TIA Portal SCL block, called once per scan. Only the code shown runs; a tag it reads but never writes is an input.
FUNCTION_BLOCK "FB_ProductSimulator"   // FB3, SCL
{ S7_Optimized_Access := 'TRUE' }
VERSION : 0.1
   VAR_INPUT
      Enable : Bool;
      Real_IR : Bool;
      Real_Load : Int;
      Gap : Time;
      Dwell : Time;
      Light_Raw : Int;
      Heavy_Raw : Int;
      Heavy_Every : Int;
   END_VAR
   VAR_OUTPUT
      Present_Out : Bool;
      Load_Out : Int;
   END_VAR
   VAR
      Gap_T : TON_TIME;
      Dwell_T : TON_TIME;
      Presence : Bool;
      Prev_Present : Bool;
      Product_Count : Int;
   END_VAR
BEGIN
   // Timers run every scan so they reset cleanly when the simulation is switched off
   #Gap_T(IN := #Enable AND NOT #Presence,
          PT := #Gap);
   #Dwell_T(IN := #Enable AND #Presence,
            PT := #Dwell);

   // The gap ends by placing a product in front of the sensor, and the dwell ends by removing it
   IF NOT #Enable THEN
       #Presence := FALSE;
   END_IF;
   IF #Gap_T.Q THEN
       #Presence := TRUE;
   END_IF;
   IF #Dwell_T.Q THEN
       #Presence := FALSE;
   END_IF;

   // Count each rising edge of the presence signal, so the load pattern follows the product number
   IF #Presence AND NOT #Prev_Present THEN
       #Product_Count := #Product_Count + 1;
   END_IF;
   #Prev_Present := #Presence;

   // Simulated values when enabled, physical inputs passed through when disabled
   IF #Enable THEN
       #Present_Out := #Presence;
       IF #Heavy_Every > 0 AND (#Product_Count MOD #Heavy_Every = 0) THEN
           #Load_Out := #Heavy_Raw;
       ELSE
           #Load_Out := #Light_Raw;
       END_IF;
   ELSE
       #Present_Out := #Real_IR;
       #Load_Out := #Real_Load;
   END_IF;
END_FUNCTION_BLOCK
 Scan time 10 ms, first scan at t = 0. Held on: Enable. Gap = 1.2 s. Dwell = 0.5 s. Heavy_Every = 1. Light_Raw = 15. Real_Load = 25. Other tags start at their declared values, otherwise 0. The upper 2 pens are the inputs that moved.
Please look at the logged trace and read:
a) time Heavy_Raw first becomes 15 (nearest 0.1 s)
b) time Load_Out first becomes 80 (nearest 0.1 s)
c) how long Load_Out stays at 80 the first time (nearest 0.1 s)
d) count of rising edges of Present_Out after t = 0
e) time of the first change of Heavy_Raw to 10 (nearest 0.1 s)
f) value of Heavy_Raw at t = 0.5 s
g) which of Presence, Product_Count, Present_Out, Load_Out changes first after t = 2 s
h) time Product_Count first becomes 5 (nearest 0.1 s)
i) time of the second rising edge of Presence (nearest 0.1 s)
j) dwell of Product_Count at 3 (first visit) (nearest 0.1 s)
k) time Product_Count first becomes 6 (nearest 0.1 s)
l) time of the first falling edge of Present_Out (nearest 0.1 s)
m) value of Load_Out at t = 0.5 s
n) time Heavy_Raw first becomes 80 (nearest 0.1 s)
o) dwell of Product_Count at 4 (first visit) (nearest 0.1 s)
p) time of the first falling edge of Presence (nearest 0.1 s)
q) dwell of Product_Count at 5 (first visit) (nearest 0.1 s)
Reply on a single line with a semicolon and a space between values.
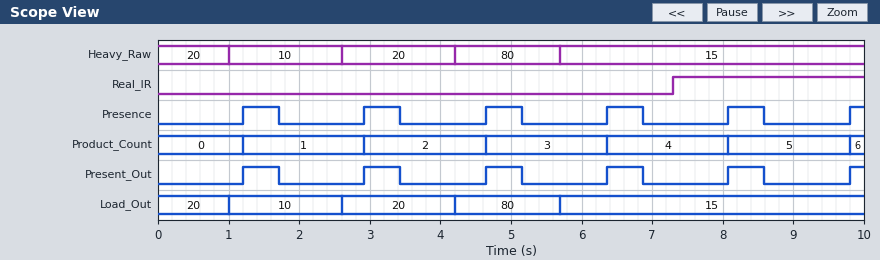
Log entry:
5.7 s; 4.2 s; 1.5 s; 6; 1.0 s; 20; Load_Out; 8.1 s; 2.9 s; 1.7 s; 9.8 s; 1.7 s; 20; 4.2 s; 1.7 s; 1.7 s; 1.7 s
